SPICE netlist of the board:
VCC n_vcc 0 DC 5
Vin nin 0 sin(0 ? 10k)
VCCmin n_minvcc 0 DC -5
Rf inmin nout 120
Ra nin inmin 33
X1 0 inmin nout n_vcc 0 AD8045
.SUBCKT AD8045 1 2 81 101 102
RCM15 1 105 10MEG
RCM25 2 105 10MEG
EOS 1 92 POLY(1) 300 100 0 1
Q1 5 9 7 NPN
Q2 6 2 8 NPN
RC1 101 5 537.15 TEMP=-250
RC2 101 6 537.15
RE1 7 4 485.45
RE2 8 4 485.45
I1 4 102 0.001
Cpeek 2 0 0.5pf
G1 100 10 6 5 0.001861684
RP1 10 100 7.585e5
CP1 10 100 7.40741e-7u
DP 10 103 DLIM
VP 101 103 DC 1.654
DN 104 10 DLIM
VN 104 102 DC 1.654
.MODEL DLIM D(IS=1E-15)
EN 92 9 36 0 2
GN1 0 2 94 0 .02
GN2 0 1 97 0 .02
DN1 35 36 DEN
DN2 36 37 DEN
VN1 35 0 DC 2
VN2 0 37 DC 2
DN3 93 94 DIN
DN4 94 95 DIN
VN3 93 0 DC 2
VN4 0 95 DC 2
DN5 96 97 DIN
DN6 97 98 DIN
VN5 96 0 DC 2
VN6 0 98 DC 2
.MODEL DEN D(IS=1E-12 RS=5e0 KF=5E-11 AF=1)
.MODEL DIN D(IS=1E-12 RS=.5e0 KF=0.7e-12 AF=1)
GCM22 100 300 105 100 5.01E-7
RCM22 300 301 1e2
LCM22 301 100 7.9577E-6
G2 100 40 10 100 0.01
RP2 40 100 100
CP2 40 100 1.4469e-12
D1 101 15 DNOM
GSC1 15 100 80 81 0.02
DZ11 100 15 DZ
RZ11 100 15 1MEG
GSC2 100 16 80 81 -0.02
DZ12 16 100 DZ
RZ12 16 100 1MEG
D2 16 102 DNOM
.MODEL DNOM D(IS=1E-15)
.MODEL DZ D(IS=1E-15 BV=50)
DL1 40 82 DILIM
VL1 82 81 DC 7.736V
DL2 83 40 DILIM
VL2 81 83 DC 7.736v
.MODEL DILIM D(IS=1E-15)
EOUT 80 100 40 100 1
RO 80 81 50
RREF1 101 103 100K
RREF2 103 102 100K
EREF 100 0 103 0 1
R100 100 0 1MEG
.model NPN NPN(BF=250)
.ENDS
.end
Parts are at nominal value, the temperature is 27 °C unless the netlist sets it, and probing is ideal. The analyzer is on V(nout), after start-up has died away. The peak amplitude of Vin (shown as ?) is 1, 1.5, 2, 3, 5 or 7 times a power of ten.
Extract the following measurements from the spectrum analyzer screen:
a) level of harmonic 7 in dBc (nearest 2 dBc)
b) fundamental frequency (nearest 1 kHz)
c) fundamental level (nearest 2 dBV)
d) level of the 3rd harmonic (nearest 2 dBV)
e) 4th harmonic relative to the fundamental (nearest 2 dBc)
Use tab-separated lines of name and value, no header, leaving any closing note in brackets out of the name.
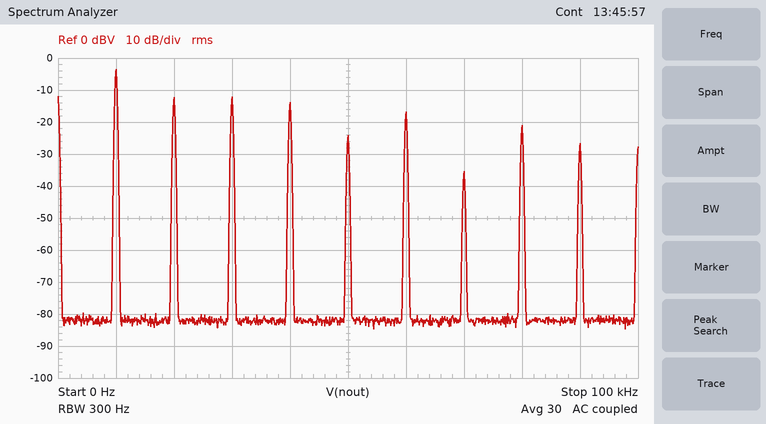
level of harmonic 7 in dBc	-32 dBc
fundamental frequency	10 kHz
fundamental level	-4 dBV
level of the 3rd harmonic	-12 dBV
4th harmonic relative to the fundamental	-10 dBc
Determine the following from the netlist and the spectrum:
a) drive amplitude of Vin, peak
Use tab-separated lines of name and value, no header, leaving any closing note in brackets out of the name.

drive amplitude of Vin, peak	2 V
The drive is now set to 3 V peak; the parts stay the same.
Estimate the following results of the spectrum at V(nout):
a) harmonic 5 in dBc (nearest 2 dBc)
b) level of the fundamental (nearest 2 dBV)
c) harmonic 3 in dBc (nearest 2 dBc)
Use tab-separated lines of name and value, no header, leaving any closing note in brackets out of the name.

harmonic 5 in dBc	-12 dBc
level of the fundamental	-6 dBV
harmonic 3 in dBc	-4 dBc
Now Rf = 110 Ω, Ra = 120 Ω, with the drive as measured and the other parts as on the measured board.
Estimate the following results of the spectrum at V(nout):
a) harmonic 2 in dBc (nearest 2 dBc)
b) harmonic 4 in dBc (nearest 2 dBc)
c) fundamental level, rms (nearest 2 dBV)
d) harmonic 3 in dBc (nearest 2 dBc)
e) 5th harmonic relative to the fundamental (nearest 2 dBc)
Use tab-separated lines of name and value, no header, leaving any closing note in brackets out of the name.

harmonic 2 in dBc	4 dBc
harmonic 4 in dBc	-24 dBc
fundamental level, rms	-14 dBV
harmonic 3 in dBc	-6 dBc
5th harmonic relative to the fundamental	-14 dBc
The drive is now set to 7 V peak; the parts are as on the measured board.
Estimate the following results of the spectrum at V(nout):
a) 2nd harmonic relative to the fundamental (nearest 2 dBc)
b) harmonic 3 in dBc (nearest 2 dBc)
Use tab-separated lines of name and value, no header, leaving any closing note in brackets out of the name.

2nd harmonic relative to the fundamental	-2 dBc
harmonic 3 in dBc	2 dBc
